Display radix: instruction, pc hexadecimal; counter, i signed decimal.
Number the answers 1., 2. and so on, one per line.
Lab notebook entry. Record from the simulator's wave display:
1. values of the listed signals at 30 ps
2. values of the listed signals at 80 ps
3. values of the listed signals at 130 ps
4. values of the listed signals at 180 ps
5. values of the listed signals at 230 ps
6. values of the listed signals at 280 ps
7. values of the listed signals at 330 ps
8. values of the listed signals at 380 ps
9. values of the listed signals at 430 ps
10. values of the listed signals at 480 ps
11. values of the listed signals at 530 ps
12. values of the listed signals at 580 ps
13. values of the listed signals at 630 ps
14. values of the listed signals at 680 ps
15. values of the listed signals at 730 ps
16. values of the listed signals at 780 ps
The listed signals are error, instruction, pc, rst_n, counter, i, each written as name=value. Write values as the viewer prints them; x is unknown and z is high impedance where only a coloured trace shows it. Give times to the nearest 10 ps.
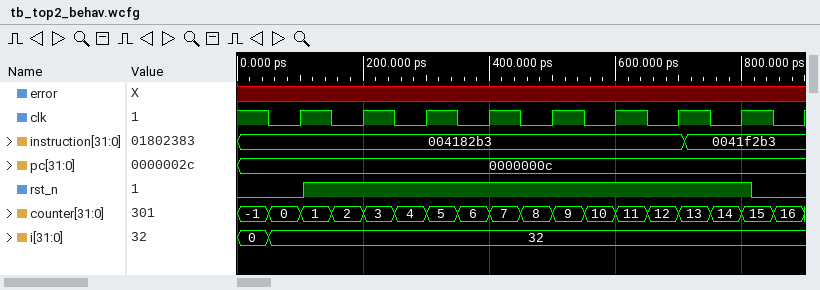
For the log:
1. error=x, instruction=004182b3, pc=0000000c, rst_n=0, counter=-1, i=0
2. error=x, instruction=004182b3, pc=0000000c, rst_n=0, counter=0, i=32
3. error=x, instruction=004182b3, pc=0000000c, rst_n=1, counter=1, i=32
4. error=x, instruction=004182b3, pc=0000000c, rst_n=1, counter=2, i=32
5. error=x, instruction=004182b3, pc=0000000c, rst_n=1, counter=3, i=32
6. error=x, instruction=004182b3, pc=0000000c, rst_n=1, counter=4, i=32
7. error=x, instruction=004182b3, pc=0000000c, rst_n=1, counter=5, i=32
8. error=x, instruction=004182b3, pc=0000000c, rst_n=1, counter=6, i=32
9. error=x, instruction=004182b3, pc=0000000c, rst_n=1, counter=7, i=32
10. error=x, instruction=004182b3, pc=0000000c, rst_n=1, counter=8, i=32
11. error=x, instruction=004182b3, pc=0000000c, rst_n=1, counter=9, i=32
12. error=x, instruction=004182b3, pc=0000000c, rst_n=1, counter=10, i=32
13. error=x, instruction=004182b3, pc=0000000c, rst_n=1, counter=11, i=32
14. error=x, instruction=004182b3, pc=0000000c, rst_n=1, counter=12, i=32
15. error=x, instruction=0041f2b3, pc=0000000c, rst_n=1, counter=13, i=32
16. error=x, instruction=0041f2b3, pc=0000000c, rst_n=1, counter=14, i=32
